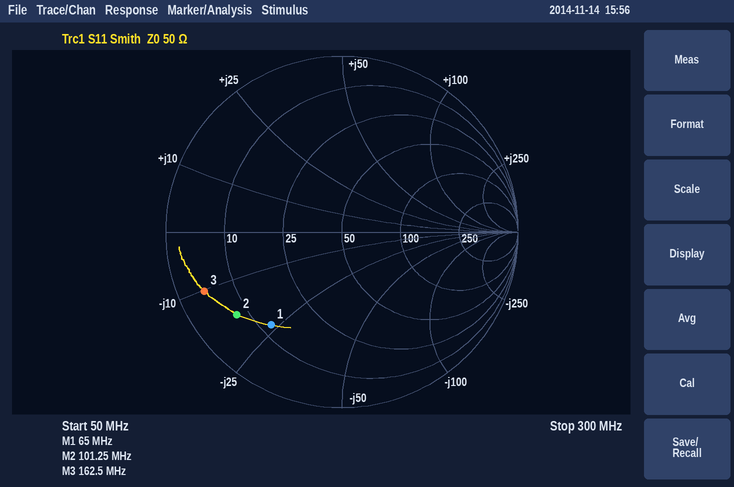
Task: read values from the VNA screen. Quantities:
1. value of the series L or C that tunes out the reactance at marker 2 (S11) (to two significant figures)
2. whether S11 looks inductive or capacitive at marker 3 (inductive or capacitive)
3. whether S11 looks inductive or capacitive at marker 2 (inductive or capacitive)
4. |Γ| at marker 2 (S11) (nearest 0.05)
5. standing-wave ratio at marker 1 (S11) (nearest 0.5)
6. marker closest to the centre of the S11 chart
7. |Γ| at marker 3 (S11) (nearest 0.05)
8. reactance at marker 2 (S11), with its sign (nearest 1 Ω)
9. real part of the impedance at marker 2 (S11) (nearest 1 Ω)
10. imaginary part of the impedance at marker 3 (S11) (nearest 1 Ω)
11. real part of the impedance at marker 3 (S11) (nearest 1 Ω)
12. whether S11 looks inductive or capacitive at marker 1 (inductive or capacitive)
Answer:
27 nH
capacitive
capacitive
0.75
5.0
marker 1
0.85
-17 Ω
8 Ω
-10 Ω
4 Ω
capacitive
